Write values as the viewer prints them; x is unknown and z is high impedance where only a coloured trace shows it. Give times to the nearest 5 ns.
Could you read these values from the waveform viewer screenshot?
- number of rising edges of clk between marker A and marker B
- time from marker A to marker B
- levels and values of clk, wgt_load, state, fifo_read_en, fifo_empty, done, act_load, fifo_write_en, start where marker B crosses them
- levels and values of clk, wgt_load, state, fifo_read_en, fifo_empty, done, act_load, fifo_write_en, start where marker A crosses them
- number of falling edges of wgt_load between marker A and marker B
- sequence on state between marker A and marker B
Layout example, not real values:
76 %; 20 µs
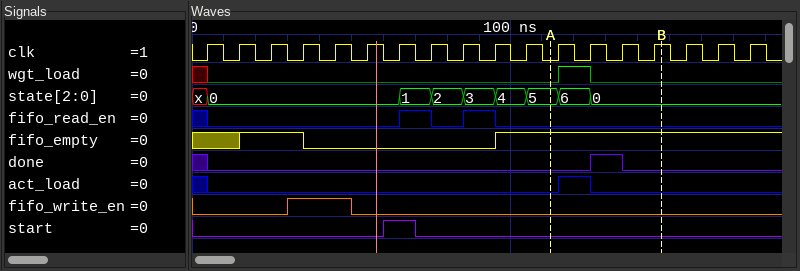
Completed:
4; 35 ns; clk=1, wgt_load=0, state=0, fifo_read_en=0, fifo_empty=1, done=0, act_load=0, fifo_write_en=0, start=0; clk=0, wgt_load=0, state=5, fifo_read_en=0, fifo_empty=1, done=0, act_load=0, fifo_write_en=0, start=0; 1; 5, 6, 0
